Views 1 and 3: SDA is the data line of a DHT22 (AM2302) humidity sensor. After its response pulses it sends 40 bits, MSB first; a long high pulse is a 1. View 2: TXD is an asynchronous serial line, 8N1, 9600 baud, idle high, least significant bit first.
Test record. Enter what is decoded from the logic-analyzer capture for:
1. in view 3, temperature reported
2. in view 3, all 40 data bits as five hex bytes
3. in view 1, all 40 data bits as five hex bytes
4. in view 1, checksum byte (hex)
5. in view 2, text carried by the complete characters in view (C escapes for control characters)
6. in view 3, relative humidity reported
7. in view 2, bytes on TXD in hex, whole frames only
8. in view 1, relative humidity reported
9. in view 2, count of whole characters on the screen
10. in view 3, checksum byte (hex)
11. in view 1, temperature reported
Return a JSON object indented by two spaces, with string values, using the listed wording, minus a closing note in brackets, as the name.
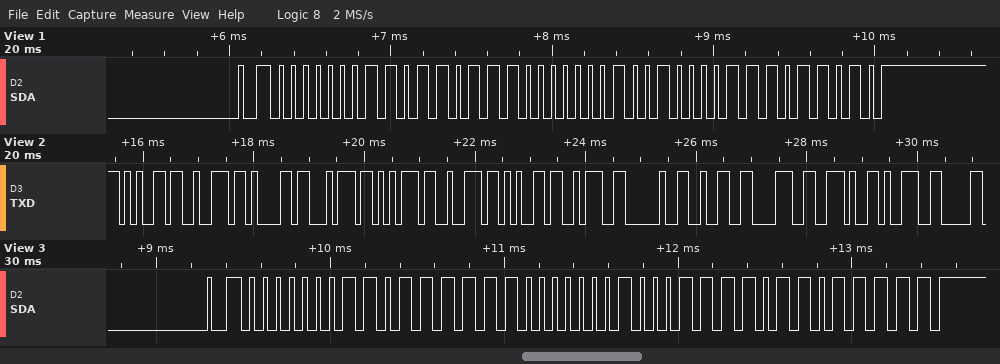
{
  "in view 3, temperature reported": "28.6 °C",
  "in view 3, all 40 data bits as five hex bytes": "01 BF 01 1E DF",
  "in view 1, all 40 data bits as five hex bytes": "01 B7 01 21 DA",
  "in view 1, checksum byte": "0xDA",
  "in view 2, text carried by the complete characters in view": "\"erature: 28.9\"",
  "in view 3, relative humidity reported": "44.7 %",
  "in view 2, bytes on TXD in hex, whole frames only": "65 72 61 74 75 72 65 3A 20 32 38 2E 39",
  "in view 1, relative humidity reported": "43.9 %",
  "in view 2, count of whole characters on the screen": "13",
  "in view 3, checksum byte": "0xDF",
  "in view 1, temperature reported": "28.9 °C"
}
